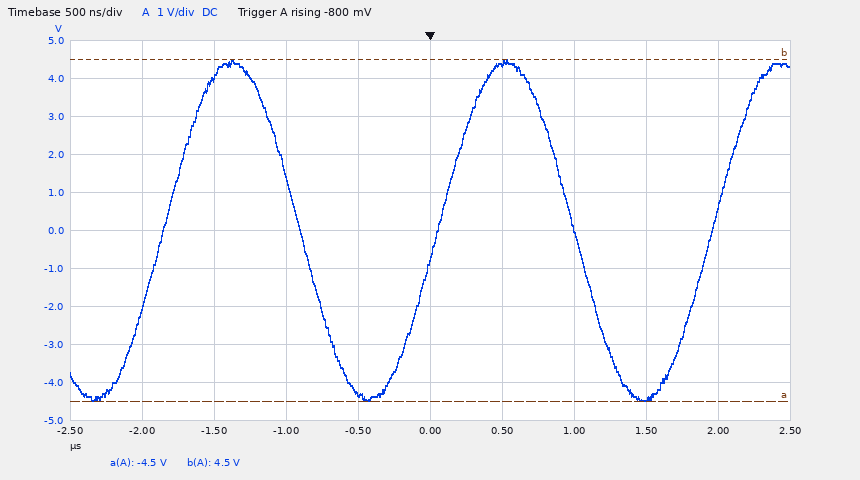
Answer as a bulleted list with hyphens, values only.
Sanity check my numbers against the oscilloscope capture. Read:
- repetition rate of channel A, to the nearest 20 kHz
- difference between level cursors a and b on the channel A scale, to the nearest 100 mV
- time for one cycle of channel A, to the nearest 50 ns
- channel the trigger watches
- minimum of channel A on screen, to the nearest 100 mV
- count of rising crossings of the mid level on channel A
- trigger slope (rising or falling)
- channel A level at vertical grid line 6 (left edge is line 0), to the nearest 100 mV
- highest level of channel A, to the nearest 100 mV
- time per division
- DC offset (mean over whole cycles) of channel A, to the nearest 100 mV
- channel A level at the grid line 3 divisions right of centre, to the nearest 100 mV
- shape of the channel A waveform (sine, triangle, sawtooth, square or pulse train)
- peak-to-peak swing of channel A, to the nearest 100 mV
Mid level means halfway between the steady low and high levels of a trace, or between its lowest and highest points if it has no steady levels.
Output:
- 520 kHz
- 9.0 V
- 1.90 µs
- channel A
- -4.5 V
- 3
- rising
- 4.4 V
- 4.5 V
- 500 ns
- 0.0 V
- -4.4 V
- sine
- 9.0 V
